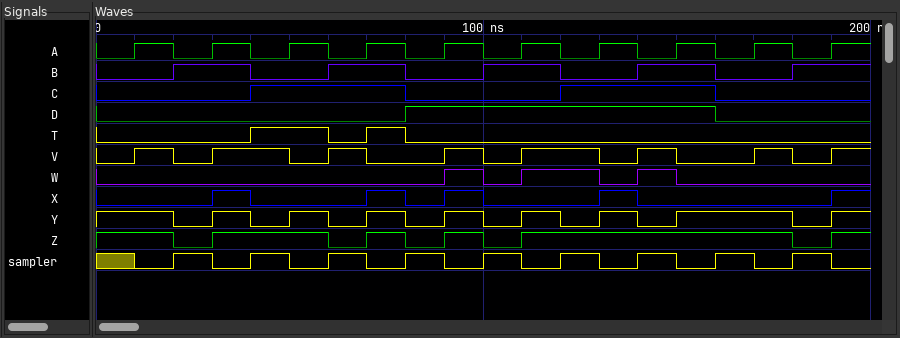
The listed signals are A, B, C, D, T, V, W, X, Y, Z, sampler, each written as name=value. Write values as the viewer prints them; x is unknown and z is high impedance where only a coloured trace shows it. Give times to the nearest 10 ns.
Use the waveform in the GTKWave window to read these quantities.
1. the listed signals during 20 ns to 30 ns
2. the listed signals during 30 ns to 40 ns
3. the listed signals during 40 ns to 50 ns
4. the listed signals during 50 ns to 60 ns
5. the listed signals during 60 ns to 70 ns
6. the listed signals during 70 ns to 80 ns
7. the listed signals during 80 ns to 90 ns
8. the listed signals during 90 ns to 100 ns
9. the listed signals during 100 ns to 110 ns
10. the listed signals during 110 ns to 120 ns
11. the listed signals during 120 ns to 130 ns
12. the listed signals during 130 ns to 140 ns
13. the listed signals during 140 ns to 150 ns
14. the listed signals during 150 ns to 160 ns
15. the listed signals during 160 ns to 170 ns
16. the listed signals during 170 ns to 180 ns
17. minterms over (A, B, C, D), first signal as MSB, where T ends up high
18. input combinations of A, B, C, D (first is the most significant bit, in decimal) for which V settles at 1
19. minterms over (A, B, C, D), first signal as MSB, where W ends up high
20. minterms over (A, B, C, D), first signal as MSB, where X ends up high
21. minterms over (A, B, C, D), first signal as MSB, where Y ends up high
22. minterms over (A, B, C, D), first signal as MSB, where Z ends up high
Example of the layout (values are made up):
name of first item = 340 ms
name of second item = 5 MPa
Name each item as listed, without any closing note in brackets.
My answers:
the listed signals during 20 ns to 30 ns = A=0, B=1, C=0, D=0, T=0, V=0, W=0, X=0, Y=0, Z=0, sampler=1
the listed signals during 30 ns to 40 ns = A=1, B=1, C=0, D=0, T=0, V=1, W=0, X=1, Y=1, Z=1, sampler=0
the listed signals during 40 ns to 50 ns = A=0, B=0, C=1, D=0, T=1, V=1, W=0, X=0, Y=0, Z=1, sampler=1
the listed signals during 50 ns to 60 ns = A=1, B=0, C=1, D=0, T=1, V=0, W=0, X=0, Y=1, Z=1, sampler=0
the listed signals during 60 ns to 70 ns = A=0, B=1, C=1, D=0, T=0, V=1, W=0, X=0, Y=0, Z=0, sampler=1
the listed signals during 70 ns to 80 ns = A=1, B=1, C=1, D=0, T=1, V=0, W=0, X=1, Y=1, Z=1, sampler=0
the listed signals during 80 ns to 90 ns = A=0, B=0, C=0, D=1, T=0, V=0, W=0, X=0, Y=0, Z=0, sampler=1
the listed signals during 90 ns to 100 ns = A=1, B=0, C=0, D=1, T=0, V=1, W=1, X=1, Y=1, Z=1, sampler=0
the listed signals during 100 ns to 110 ns = A=0, B=1, C=0, D=1, T=0, V=0, W=0, X=0, Y=0, Z=0, sampler=1
the listed signals during 110 ns to 120 ns = A=1, B=1, C=0, D=1, T=0, V=1, W=1, X=0, Y=1, Z=1, sampler=0
the listed signals during 120 ns to 130 ns = A=0, B=0, C=1, D=1, T=0, V=1, W=1, X=0, Y=0, Z=1, sampler=1
the listed signals during 130 ns to 140 ns = A=1, B=0, C=1, D=1, T=0, V=0, W=0, X=1, Y=1, Z=1, sampler=0
the listed signals during 140 ns to 150 ns = A=0, B=1, C=1, D=1, T=0, V=1, W=1, X=0, Y=0, Z=1, sampler=1
the listed signals during 150 ns to 160 ns = A=1, B=1, C=1, D=1, T=0, V=0, W=0, X=0, Y=1, Z=1, sampler=0
the listed signals during 160 ns to 170 ns = A=0, B=0, C=0, D=0, T=0, V=0, W=0, X=0, Y=1, Z=1, sampler=1
the listed signals during 170 ns to 180 ns = A=1, B=0, C=0, D=0, T=0, V=1, W=0, X=0, Y=1, Z=1, sampler=0
minterms over (A, B, C, D), first signal as MSB, where T ends up high = 2, 10, 14
input combinations of A, B, C, D (first is the most significant bit, in decimal) for which V settles at 1 = 2, 3, 6, 7, 8, 9, 12, 13
minterms over (A, B, C, D), first signal as MSB, where W ends up high = 3, 7, 9, 13
minterms over (A, B, C, D), first signal as MSB, where X ends up high = 9, 11, 12, 14
minterms over (A, B, C, D), first signal as MSB, where Y ends up high = 0, 8, 9, 10, 11, 12, 13, 14, 15
minterms over (A, B, C, D), first signal as MSB, where Z ends up high = 0, 2, 3, 7, 8, 9, 10, 11, 12, 13, 14, 15
